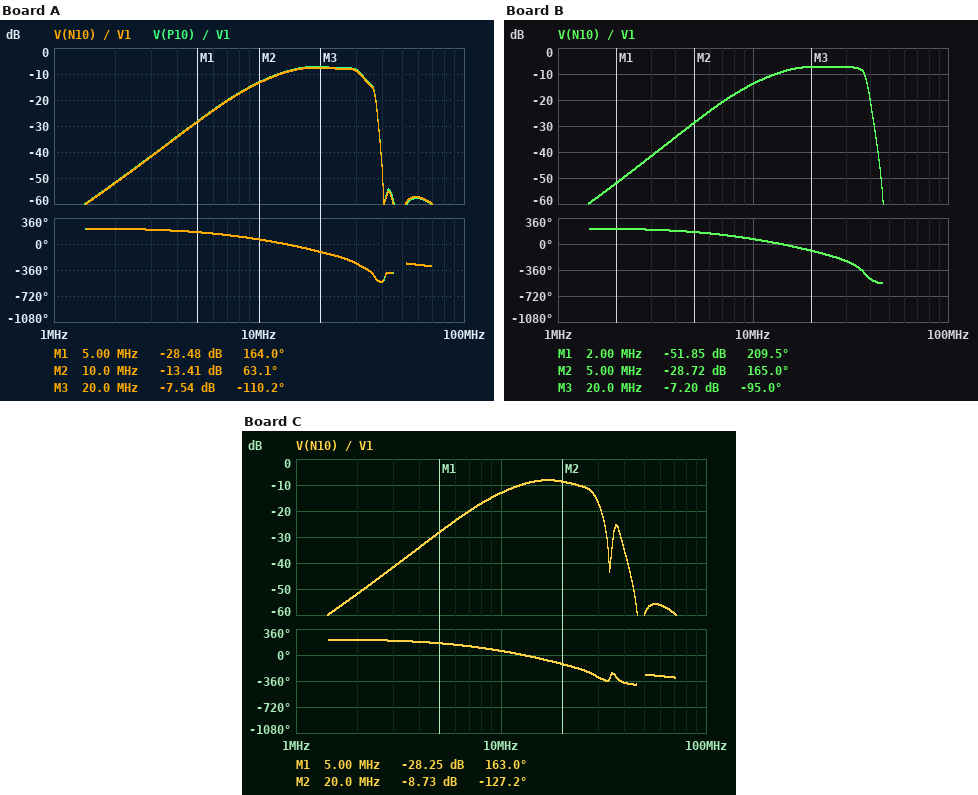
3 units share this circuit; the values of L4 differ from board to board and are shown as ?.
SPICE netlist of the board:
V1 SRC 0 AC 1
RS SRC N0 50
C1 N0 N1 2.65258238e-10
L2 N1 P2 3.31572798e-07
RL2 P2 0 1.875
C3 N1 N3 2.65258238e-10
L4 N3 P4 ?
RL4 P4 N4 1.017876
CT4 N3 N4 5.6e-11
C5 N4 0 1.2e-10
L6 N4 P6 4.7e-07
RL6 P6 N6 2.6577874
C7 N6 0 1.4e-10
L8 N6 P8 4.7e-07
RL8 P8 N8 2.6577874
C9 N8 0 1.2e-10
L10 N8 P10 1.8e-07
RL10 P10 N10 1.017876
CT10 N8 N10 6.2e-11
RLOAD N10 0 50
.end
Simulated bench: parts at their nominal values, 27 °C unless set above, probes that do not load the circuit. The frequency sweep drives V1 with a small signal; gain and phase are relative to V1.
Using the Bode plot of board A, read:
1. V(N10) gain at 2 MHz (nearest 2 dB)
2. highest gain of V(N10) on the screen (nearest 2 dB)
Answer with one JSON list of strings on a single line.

["-52 dB", "-8 dB"]
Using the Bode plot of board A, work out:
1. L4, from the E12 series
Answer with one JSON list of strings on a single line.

["270 nH"]
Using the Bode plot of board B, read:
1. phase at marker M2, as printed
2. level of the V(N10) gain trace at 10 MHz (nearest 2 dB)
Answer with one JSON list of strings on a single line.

["165.0 deg", "-14 dB"]
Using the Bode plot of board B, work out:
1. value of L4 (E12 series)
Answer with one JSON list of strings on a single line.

["150 nH"]
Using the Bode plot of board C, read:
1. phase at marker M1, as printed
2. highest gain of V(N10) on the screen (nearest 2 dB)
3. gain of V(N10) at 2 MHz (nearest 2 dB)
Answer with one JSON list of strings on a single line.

["163.0 deg", "-8 dB", "-52 dB"]
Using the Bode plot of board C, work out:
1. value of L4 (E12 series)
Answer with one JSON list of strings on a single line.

["390 nH"]
